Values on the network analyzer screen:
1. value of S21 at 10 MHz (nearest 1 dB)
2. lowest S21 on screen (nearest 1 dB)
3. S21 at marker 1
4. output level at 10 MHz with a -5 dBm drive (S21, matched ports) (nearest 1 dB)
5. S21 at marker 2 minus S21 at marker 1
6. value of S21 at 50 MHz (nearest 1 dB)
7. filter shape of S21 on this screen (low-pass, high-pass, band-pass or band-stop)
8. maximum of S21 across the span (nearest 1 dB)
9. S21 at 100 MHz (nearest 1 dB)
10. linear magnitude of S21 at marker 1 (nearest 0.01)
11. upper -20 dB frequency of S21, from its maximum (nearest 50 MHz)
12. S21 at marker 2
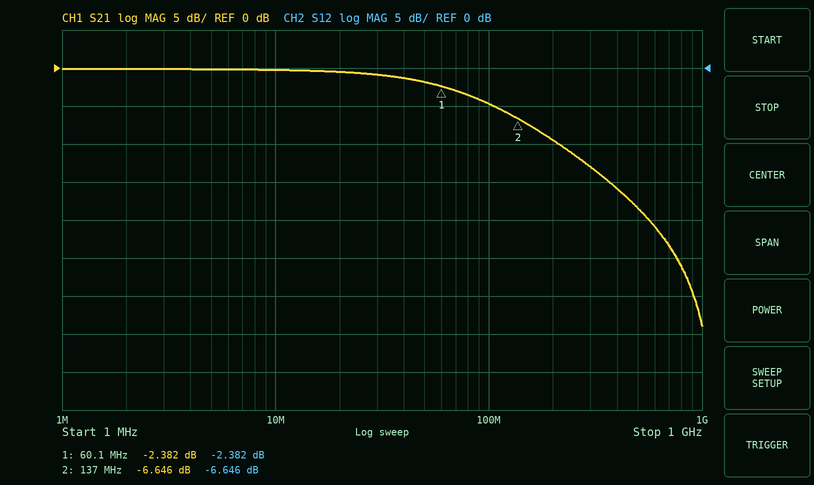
0 dB
-34 dB
-2.382 dB
-5 dBm
-4.264 dB
-2 dB
low-pass
0 dB
-5 dB
0.76
550 MHz
-6.646 dB
